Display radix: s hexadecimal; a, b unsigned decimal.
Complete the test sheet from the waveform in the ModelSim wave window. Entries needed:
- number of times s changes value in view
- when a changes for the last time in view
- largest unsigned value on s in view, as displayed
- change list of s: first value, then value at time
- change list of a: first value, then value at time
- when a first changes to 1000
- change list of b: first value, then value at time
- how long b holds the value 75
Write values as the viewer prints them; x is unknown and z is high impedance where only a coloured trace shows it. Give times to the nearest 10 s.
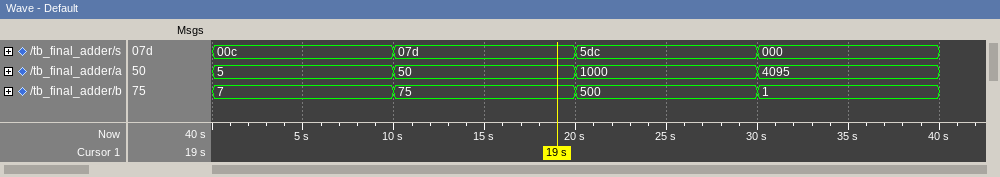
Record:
3
30 s
5dc
00c, 07d at 10 s, 5dc at 20 s, 000 at 30 s
5, 50 at 10 s, 1000 at 20 s, 4095 at 30 s
20 s
7, 75 at 10 s, 500 at 20 s, 1 at 30 s
10 s
